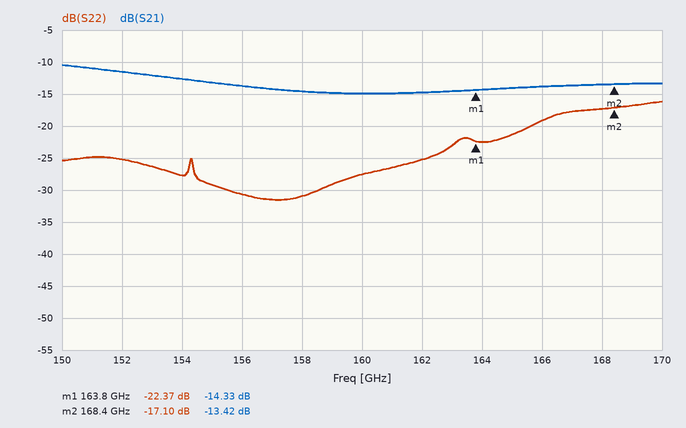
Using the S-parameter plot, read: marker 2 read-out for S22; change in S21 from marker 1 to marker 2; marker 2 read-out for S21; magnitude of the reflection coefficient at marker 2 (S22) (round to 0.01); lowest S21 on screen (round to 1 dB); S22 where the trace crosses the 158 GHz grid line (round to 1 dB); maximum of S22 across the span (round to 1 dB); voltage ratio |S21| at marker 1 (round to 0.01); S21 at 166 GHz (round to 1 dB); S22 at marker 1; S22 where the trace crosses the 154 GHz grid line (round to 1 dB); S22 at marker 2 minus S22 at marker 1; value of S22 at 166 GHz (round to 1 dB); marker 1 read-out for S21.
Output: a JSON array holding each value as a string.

["-17.10 dB", "0.91 dB", "-13.42 dB", "0.14", "-15 dB", "-31 dB", "-16 dB", "0.19", "-14 dB", "-22.37 dB", "-28 dB", "5.27 dB", "-19 dB", "-14.33 dB"]
